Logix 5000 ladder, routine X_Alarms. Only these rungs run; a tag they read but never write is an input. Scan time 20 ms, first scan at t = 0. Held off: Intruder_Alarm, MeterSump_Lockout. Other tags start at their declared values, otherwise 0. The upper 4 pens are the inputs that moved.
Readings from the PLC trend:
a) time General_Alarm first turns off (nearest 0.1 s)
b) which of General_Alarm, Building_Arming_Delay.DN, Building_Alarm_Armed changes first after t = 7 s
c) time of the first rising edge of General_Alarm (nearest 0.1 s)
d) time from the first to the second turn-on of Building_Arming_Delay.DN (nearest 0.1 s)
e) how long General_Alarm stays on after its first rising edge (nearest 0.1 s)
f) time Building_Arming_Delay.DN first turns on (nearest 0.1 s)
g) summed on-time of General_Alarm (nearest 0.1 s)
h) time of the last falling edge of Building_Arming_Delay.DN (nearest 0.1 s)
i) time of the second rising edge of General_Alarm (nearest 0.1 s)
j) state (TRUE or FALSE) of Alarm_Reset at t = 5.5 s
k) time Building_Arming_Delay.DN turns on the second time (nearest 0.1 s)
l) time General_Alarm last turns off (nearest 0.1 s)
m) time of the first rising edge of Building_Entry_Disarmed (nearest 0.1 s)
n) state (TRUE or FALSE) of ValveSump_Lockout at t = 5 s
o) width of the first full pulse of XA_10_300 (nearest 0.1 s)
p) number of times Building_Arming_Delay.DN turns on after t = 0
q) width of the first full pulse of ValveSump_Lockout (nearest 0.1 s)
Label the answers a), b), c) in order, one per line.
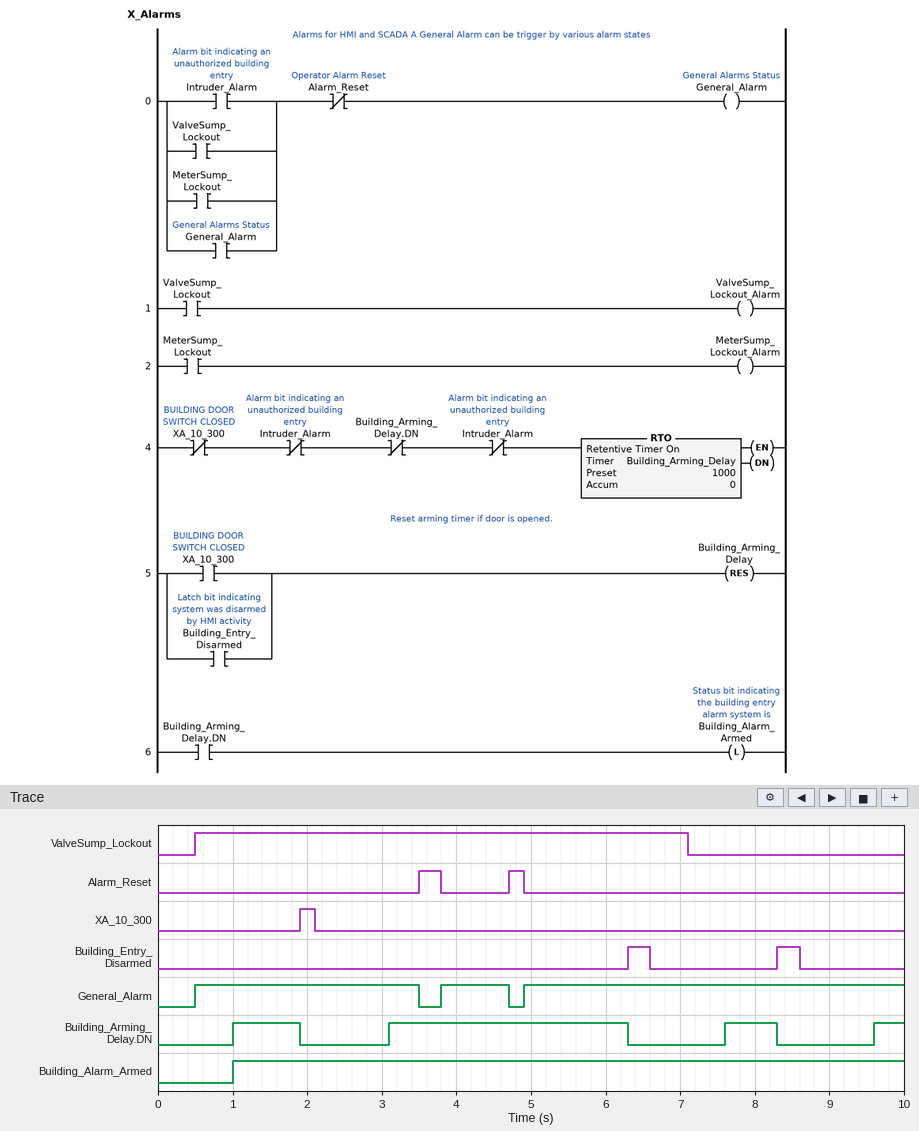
a) 3.5 s
b) Building_Arming_Delay.DN
c) 0.5 s
d) 2.1 s
e) 3.0 s
f) 1.0 s
g) 9.0 s
h) 8.3 s
i) 3.8 s
j) FALSE
k) 3.1 s
l) 4.7 s
m) 6.3 s
n) TRUE
o) 0.2 s
p) 4
q) 6.6 s
